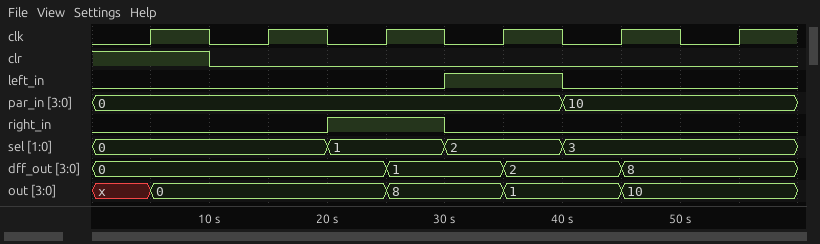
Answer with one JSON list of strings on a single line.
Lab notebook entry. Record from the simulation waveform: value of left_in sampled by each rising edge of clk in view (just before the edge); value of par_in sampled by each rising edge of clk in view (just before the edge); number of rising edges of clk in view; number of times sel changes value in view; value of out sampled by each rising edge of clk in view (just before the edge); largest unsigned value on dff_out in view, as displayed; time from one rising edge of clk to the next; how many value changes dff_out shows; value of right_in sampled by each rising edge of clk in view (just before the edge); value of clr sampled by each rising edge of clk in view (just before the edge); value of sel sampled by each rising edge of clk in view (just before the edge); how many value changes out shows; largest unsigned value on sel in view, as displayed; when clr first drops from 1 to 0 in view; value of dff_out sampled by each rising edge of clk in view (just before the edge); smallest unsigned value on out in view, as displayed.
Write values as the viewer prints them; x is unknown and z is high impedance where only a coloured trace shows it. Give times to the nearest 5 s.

["0 0 0 1 0 0", "0, 0, 0, 0, 10, 10", "6", "3", "x, 0, 0, 8, 1, 10", "8", "10 s", "3", "0 0 1 0 0 0", "1 0 0 0 0 0", "0, 0, 1, 2, 3, 3", "4", "3", "10 s", "0, 0, 0, 1, 2, 8", "0"]
